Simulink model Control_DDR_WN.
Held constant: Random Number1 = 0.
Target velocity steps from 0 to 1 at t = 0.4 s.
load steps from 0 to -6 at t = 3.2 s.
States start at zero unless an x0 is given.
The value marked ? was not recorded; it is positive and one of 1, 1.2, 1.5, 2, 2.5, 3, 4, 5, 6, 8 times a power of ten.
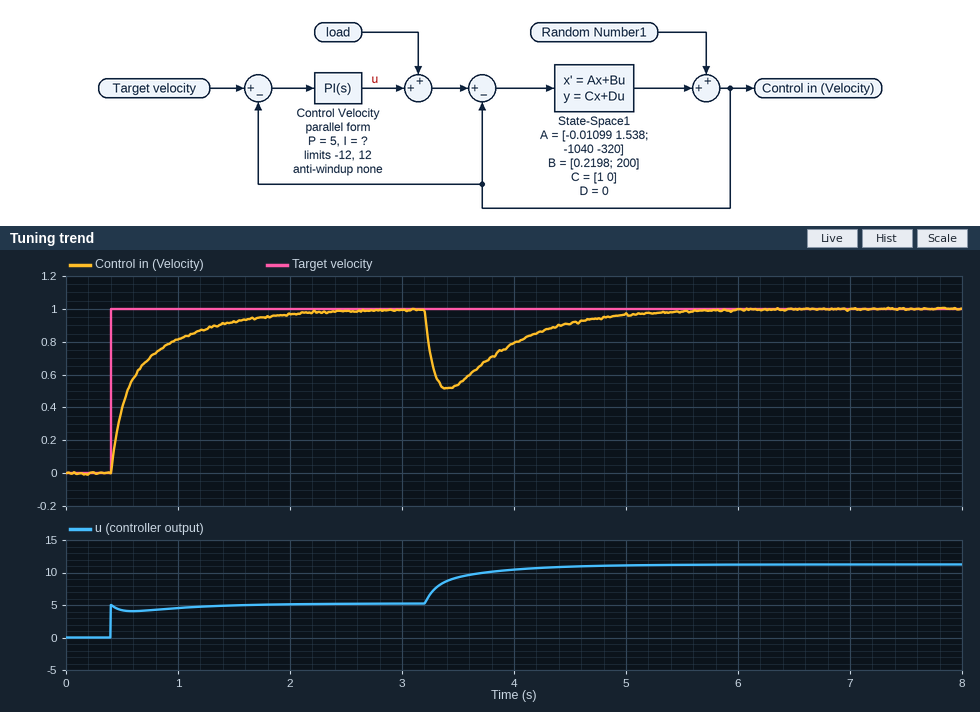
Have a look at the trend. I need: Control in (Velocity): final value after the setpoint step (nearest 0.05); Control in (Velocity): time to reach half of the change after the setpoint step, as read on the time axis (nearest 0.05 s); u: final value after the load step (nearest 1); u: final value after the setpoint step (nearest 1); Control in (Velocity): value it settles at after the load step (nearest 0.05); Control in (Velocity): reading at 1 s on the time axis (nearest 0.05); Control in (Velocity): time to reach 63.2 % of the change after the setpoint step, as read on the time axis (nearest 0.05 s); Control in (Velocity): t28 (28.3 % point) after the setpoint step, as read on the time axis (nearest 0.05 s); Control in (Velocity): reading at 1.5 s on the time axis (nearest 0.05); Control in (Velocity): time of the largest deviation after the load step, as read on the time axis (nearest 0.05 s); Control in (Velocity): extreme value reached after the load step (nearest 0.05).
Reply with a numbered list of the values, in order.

1. 1.00
2. 0.55 s
3. 11
4. 5
5. 1.00
6. 0.80
7. 0.65 s
8. 0.45 s
9. 0.90
10. 3.40 s
11. 0.50
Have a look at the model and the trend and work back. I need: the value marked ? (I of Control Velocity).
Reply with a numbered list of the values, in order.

1. 15
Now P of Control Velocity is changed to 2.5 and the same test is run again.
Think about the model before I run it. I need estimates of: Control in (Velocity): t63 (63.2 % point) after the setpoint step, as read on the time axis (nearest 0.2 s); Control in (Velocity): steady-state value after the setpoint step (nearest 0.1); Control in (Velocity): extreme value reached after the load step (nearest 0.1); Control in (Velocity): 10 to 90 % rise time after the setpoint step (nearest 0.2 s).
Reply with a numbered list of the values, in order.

1. 0.8 s
2. 1.0
3. 0.4
4. 0.8 s
